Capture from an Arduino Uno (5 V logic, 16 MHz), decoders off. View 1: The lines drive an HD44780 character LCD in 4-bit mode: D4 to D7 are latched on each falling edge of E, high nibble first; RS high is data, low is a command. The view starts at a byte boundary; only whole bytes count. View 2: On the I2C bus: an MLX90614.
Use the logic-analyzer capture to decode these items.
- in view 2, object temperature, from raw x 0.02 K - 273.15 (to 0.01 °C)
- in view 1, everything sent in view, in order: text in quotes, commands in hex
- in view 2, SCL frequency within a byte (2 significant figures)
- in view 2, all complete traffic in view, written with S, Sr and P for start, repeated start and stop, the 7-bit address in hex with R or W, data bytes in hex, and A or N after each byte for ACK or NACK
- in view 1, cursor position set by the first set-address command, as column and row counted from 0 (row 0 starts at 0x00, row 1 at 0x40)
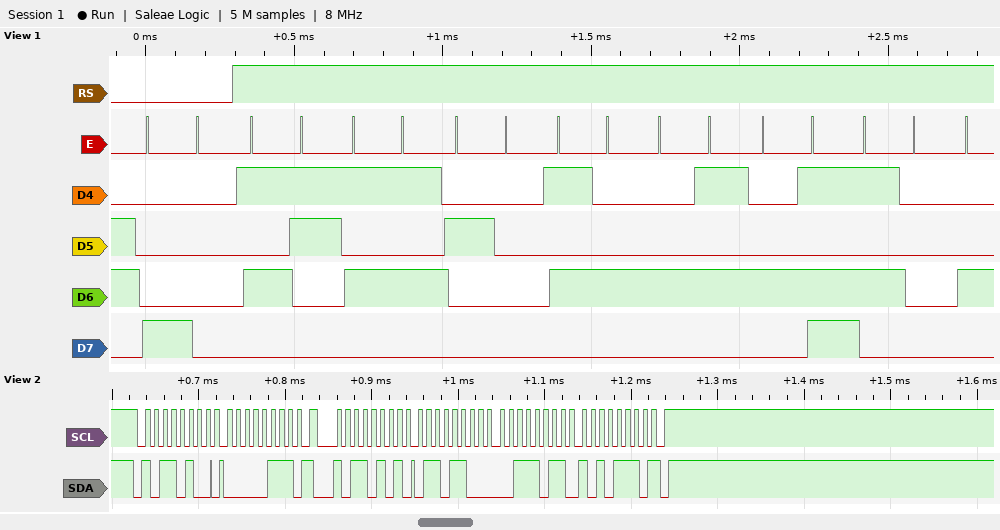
31.09 °C
0x80 "SU TEMP"
100 kHz
S 5AW A 07 A Sr 5AR A 6C A 3B A AE N P
column 0, row 0
